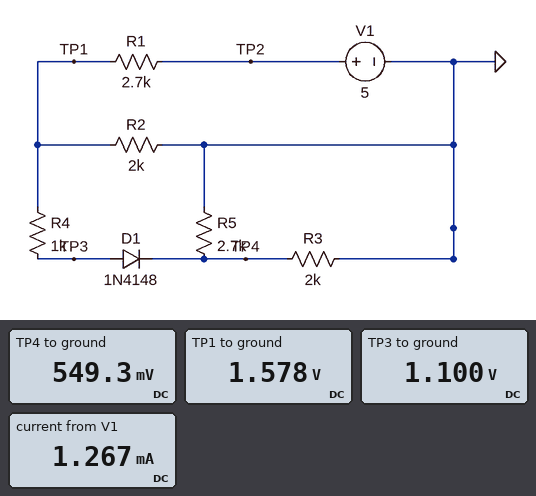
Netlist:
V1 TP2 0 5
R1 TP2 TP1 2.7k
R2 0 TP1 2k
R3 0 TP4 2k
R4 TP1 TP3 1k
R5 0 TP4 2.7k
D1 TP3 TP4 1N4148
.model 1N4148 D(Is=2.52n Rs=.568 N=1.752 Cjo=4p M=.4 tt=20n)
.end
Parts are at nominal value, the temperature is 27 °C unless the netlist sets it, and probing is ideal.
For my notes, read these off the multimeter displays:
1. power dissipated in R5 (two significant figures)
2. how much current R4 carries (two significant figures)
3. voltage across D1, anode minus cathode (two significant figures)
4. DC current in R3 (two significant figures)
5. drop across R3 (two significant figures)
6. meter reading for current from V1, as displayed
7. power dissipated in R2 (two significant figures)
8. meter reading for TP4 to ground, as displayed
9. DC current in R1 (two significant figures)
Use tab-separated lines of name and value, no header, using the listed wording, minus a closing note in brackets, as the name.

power dissipated in R5	110 µW
how much current R4 carries	480 µA
voltage across D1, anode minus cathode	550 mV
DC current in R3	270 µA
drop across R3	550 mV
meter reading for current from V1, as displayed	1.267 mA
power dissipated in R2	1.2 mW
meter reading for TP4 to ground, as displayed	549.3 mV
DC current in R1	1.3 mA
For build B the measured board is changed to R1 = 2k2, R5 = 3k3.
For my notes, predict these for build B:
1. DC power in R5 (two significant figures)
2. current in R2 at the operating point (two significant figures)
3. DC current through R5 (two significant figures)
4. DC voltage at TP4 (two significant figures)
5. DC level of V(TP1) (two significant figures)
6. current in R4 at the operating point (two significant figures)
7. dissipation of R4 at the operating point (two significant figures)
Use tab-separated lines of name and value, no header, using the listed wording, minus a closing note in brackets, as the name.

DC power in R5	140 µW
current in R2 at the operating point	900 µA
DC current through R5	210 µA
DC voltage at TP4	690 mV
DC level of V(TP1)	1.8 V
current in R4 at the operating point	550 µA
dissipation of R4 at the operating point	310 µW
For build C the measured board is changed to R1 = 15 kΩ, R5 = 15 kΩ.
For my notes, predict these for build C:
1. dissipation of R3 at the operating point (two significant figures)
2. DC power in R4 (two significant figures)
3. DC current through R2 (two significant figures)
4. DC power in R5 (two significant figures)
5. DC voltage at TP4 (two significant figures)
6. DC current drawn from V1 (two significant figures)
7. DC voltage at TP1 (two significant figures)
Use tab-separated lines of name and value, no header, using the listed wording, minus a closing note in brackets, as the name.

dissipation of R3 at the operating point	1.9 µW
DC power in R4	1.2 µW
DC current through R2	260 µA
DC power in R5	250 nW
DC voltage at TP4	61 mV
DC current drawn from V1	300 µA
DC voltage at TP1	530 mV
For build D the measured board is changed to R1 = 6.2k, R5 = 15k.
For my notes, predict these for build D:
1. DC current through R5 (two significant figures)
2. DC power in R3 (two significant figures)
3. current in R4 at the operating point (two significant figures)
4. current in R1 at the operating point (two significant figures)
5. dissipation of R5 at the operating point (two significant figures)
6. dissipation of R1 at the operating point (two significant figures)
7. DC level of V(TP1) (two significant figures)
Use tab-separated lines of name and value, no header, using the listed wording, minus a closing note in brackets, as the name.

DC current through R5	20 µA
DC power in R3	44 µW
current in R4 at the operating point	170 µA
current in R1 at the operating point	650 µA
dissipation of R5 at the operating point	5.8 µW
dissipation of R1 at the operating point	2.6 mW
DC level of V(TP1)	970 mV
